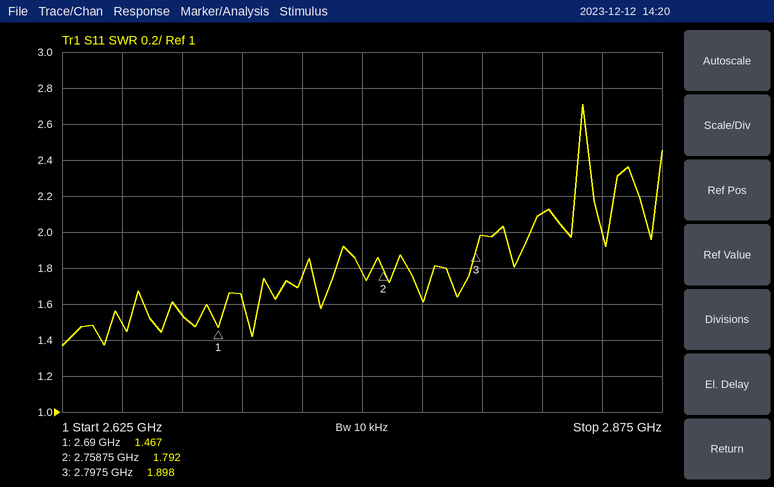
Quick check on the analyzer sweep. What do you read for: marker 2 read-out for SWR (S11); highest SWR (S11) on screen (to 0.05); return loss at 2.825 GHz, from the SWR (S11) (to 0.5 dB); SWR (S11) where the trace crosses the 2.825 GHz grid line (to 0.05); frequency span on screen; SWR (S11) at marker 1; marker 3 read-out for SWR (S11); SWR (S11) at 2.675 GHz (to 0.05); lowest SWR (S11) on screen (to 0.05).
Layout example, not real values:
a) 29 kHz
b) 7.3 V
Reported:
a) 1.792
b) 2.70
c) 9.0 dB
d) 2.10
e) 250 MHz
f) 1.467
g) 1.898
h) 1.55
i) 1.35
